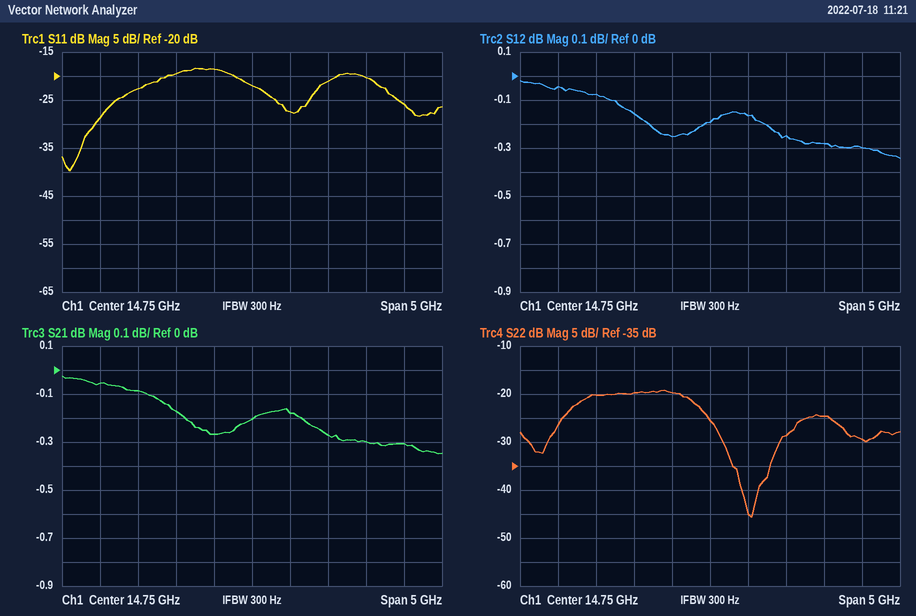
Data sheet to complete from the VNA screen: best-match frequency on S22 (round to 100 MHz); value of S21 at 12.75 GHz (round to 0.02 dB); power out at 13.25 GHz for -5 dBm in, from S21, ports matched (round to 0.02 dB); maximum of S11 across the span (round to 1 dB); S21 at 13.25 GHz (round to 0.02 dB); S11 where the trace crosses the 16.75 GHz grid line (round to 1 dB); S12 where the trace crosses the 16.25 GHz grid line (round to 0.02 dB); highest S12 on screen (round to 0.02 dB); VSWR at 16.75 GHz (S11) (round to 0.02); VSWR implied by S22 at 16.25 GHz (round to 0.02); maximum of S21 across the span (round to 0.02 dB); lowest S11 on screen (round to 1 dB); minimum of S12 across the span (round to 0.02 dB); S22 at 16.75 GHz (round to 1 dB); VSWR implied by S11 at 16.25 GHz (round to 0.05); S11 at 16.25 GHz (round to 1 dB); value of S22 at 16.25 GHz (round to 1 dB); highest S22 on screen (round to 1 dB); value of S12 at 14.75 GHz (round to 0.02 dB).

15.3 GHz
-0.06 dB
-5.08 dBm
-18 dB
-0.08 dB
-26 dB
-0.28 dB
-0.02 dB
1.10
1.12
-0.02 dB
-40 dB
-0.34 dB
-29 dB
1.20
-20 dB
-25 dB
-19 dB
-0.20 dB
